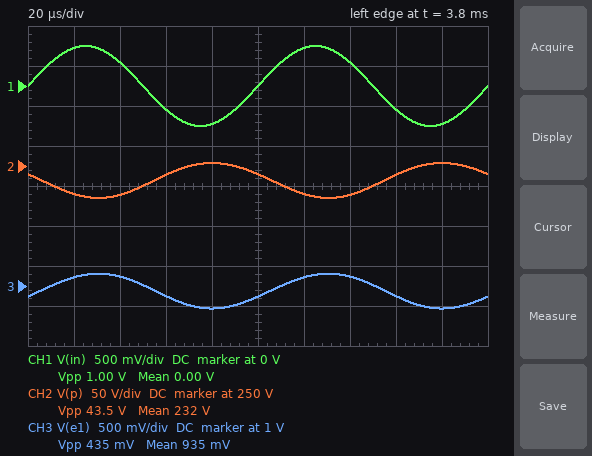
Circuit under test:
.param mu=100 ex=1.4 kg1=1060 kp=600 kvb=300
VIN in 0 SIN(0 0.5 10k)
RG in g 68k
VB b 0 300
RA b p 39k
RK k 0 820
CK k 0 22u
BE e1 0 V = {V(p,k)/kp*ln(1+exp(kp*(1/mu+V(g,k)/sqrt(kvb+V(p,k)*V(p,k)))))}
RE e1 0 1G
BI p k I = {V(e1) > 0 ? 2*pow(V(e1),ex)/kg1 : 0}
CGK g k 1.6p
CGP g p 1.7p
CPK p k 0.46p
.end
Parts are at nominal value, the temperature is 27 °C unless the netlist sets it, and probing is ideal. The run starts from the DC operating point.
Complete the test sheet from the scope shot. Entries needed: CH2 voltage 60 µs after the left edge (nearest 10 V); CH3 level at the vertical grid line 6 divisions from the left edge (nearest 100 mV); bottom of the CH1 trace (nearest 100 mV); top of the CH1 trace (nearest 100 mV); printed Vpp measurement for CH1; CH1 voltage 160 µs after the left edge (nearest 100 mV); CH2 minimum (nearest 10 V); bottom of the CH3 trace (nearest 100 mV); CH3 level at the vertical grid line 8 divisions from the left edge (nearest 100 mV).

240 V
1.1 V
-500 mV
500 mV
1.00 V
-300 mV
210 V
700 mV
900 mV
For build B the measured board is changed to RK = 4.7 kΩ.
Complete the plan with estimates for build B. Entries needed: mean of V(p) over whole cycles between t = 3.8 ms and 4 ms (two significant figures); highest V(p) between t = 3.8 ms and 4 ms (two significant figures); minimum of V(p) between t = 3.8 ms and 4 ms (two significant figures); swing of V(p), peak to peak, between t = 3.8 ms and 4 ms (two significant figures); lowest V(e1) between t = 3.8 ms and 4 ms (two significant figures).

280 V
290 V
260 V
27 V
240 mV
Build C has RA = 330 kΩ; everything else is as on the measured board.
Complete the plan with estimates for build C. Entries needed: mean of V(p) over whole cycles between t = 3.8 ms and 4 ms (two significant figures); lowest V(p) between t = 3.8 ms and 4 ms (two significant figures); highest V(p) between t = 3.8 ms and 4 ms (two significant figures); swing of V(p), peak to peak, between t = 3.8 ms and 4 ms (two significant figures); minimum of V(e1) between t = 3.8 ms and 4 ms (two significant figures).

95 V
59 V
130 V
70 V
400 mV
